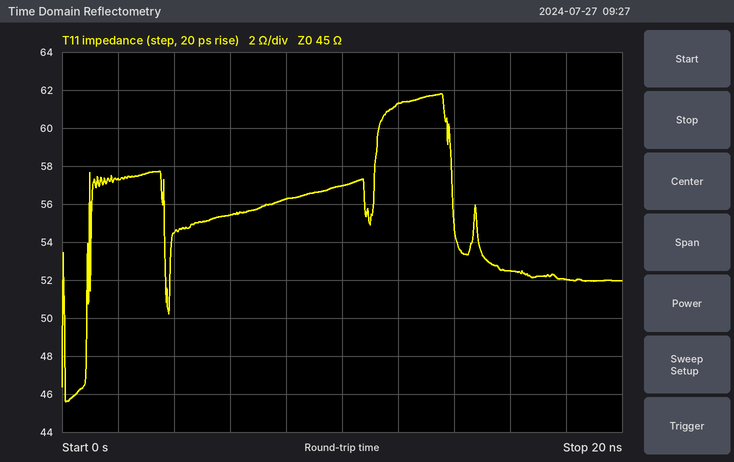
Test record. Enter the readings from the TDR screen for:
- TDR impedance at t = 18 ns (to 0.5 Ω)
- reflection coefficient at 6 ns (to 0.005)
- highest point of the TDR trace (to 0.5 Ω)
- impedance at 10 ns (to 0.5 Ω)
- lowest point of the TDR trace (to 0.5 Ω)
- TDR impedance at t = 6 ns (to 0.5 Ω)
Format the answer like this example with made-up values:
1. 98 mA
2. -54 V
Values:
1. 52.0 Ω
2. +0.105
3. 62.0 Ω
4. 57.0 Ω
5. 45.5 Ω
6. 55.5 Ω
